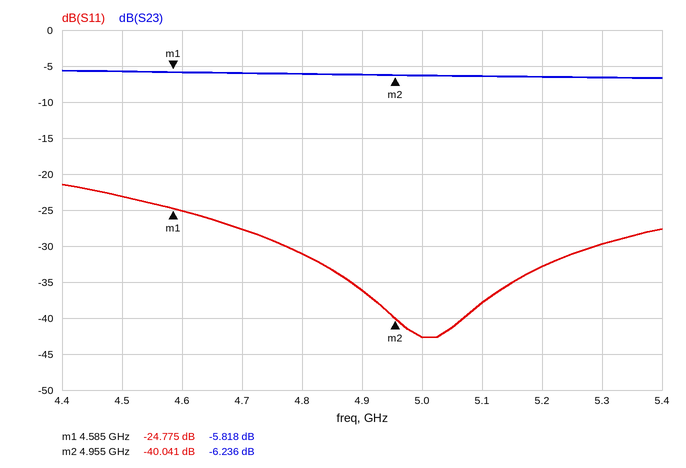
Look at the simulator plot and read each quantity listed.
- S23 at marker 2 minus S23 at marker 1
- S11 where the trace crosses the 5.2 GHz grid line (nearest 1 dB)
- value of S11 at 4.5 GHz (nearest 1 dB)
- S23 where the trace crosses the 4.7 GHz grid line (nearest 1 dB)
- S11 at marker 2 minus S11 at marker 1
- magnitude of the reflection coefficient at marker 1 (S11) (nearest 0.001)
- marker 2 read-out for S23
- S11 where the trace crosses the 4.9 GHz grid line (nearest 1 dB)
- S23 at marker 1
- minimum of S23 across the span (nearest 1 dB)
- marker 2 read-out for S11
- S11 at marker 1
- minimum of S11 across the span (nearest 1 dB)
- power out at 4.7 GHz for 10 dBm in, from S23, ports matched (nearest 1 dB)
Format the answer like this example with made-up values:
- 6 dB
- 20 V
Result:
- -0.418 dB
- -33 dB
- -23 dB
- -6 dB
- -15.266 dB
- 0.058
- -6.236 dB
- -36 dB
- -5.818 dB
- -7 dB
- -40.041 dB
- -24.775 dB
- -43 dB
- 4 dBm
